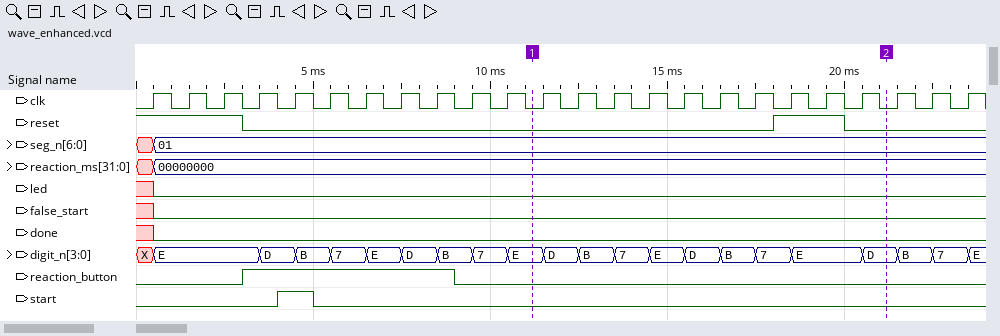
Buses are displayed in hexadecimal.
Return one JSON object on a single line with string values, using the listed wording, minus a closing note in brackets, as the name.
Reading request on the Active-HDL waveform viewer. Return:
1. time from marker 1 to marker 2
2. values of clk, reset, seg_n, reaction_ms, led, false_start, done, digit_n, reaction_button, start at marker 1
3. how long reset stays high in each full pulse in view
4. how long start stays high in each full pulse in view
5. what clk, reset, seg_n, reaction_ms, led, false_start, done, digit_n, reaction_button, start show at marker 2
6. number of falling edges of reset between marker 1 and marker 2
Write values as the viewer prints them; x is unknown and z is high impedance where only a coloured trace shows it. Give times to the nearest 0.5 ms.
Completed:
{"time from marker 1 to marker 2": "10 ms", "values of clk, reset, seg_n, reaction_ms, led, false_start, done, digit_n, reaction_button, start at marker 1": "clk=0, reset=0, seg_n=01, reaction_ms=00000000, led=0, false_start=0, done=0, digit_n=E, reaction_button=0, start=0", "how long reset stays high in each full pulse in view": "2 ms", "how long start stays high in each full pulse in view": "1 ms", "what clk, reset, seg_n, reaction_ms, led, false_start, done, digit_n, reaction_button, start show at marker 2": "clk=0, reset=0, seg_n=01, reaction_ms=00000000, led=0, false_start=0, done=0, digit_n=D, reaction_button=0, start=0", "number of falling edges of reset between marker 1 and marker 2": "1"}
